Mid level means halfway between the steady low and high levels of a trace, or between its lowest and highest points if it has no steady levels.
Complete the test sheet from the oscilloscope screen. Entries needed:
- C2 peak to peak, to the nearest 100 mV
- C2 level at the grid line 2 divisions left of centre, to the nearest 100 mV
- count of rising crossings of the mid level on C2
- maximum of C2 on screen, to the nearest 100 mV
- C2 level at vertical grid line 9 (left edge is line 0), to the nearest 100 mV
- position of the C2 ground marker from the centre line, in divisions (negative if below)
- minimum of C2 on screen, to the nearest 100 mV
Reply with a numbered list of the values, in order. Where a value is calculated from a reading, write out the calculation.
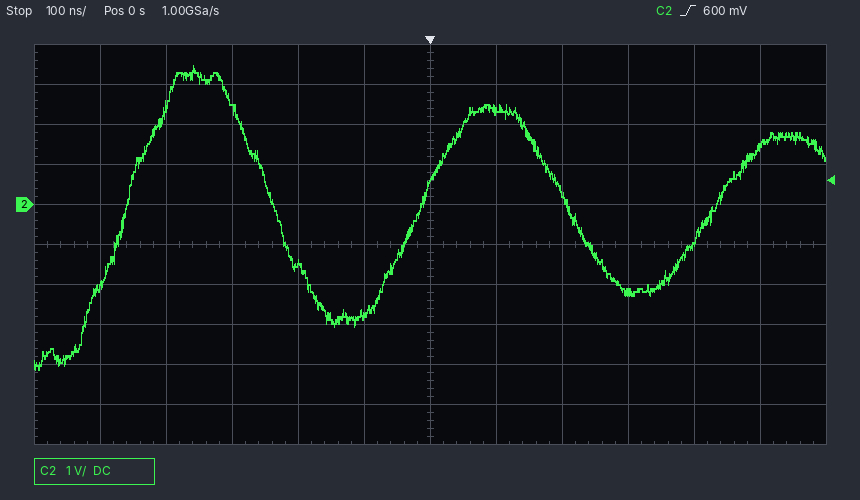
1. 3.5 V − (-4.1 V) = 7.6 V
2. -1.5 V
3. 3
4. 3.5 V
5. -2.2 V
6. +1.0 div
7. -4.1 V
